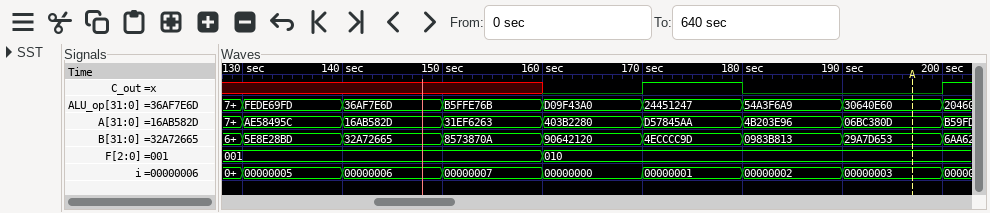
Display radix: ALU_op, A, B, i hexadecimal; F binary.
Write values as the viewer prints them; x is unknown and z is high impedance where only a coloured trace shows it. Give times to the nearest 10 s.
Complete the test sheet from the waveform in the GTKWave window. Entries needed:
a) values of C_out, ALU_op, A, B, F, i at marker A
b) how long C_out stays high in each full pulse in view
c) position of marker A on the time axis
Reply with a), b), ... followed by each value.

a) C_out=0, ALU_op=30640E60, A=06BC380D, B=29A7D653, F=010, i=00000003
b) 10 s
c) 200 s
